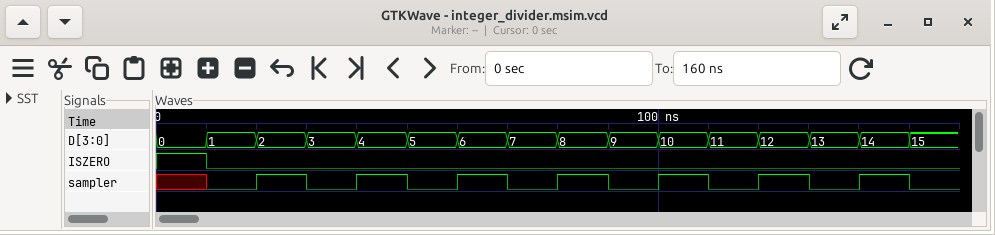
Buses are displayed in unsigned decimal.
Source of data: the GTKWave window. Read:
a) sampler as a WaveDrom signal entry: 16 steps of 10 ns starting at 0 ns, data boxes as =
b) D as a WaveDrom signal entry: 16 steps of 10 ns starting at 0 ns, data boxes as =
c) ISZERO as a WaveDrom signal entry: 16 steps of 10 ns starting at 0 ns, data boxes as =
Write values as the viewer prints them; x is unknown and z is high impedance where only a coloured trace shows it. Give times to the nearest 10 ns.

{name: 'sampler', wave: 'x010101010101010'}
{name: 'D', wave: '================', data: '0 1 2 3 4 5 6 7 8 9 10 11 12 13 14 15'}
{name: 'ISZERO', wave: '10..............'}
